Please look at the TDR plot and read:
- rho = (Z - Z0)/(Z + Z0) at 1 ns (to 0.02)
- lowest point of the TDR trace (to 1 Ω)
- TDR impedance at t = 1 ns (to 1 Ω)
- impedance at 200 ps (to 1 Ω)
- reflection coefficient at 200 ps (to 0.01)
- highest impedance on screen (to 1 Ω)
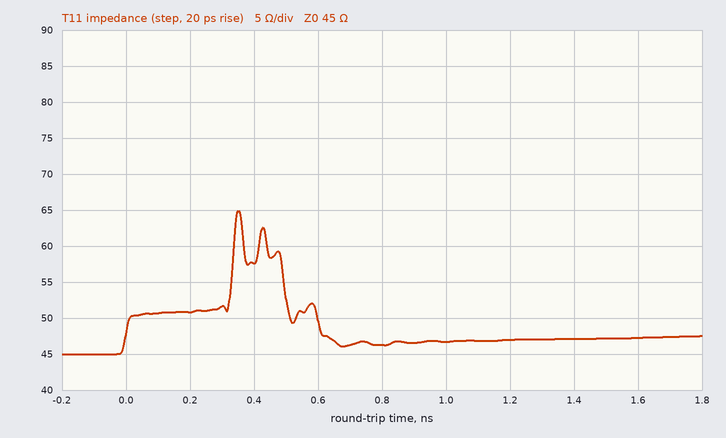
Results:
+0.02
45 Ω
47 Ω
51 Ω
+0.06
65 Ω
